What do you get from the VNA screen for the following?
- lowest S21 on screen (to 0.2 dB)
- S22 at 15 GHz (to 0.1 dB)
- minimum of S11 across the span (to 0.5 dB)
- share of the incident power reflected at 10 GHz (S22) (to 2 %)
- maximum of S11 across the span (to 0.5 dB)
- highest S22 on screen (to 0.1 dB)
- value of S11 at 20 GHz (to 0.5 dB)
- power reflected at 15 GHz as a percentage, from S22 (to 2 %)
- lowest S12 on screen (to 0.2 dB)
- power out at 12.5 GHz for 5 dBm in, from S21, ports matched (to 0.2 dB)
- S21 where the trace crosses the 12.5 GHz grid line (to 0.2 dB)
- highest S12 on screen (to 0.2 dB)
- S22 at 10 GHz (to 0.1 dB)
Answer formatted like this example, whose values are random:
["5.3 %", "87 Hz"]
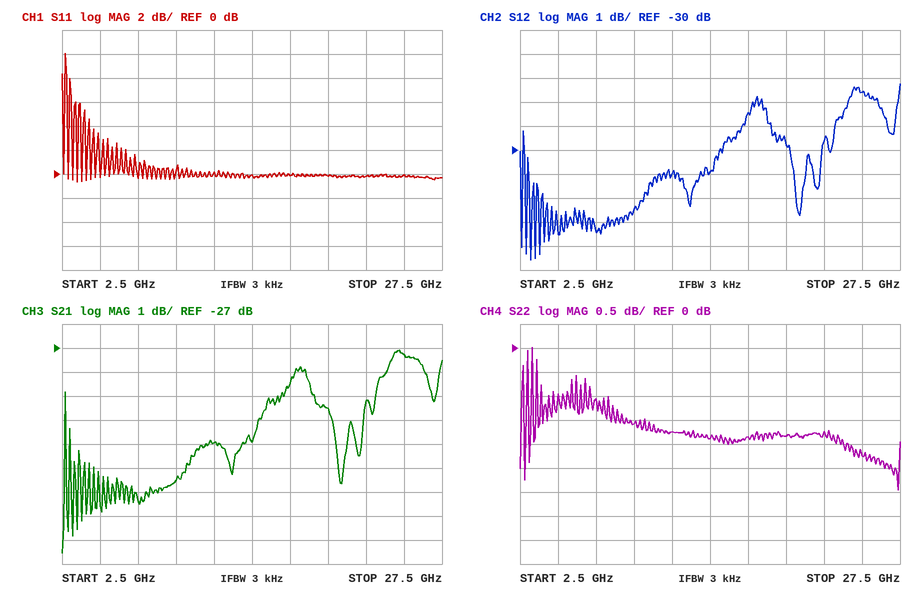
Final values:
["-35.6 dB", "-1.9 dB", "-0.5 dB", "70 %", "10.0 dB", "0.0 dB", "0.0 dB", "64 %", "-34.6 dB", "-26.0 dBm", "-31.0 dB", "-27.2 dB", "-1.6 dB"]
